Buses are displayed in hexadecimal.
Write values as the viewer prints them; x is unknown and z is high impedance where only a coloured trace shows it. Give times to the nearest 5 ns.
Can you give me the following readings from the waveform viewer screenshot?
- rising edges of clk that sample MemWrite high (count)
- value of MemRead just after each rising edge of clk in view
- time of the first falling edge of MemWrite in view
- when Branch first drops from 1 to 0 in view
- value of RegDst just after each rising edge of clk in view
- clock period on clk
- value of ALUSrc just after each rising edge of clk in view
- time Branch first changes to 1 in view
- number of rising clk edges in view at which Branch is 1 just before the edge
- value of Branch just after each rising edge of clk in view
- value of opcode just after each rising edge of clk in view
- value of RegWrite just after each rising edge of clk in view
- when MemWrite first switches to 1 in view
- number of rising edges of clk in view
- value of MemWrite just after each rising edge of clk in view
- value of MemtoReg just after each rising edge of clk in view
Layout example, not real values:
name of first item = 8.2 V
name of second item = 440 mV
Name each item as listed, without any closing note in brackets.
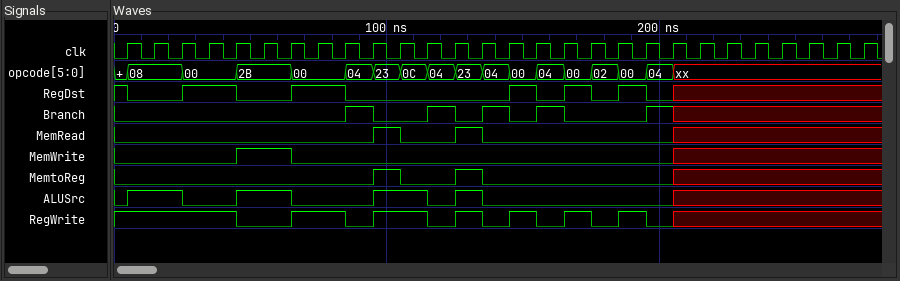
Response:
rising edges of clk that sample MemWrite high = 2
value of MemRead just after each rising edge of clk in view = 0 0 0 0 0 0 0 0 0 1 0 0 1 0 0 0 0 0 0 0 x x x x x x x x
time of the first falling edge of MemWrite in view = 65 ns
when Branch first drops from 1 to 0 in view = 95 ns
value of RegDst just after each rising edge of clk in view = 0 0 1 1 0 0 1 1 0 0 0 0 0 0 1 0 1 0 1 0 x x x x x x x x
clock period on clk = 10 ns
value of ALUSrc just after each rising edge of clk in view = 1 1 0 0 1 1 0 0 0 1 1 0 1 0 0 0 0 0 0 0 x x x x x x x x
time Branch first changes to 1 in view = 85 ns
number of rising clk edges in view at which Branch is 1 just before the edge = 5
value of Branch just after each rising edge of clk in view = 0 0 0 0 0 0 0 0 1 0 0 1 0 1 0 1 0 0 0 1 x x x x x x x x
value of opcode just after each rising edge of clk in view = 08, 08, 00, 00, 2B, 2B, 00, 00, 04, 23, 0C, 04, 23, 04, 00, 04, 00, 02, 00, 04, xx, xx, xx, xx, xx, xx, xx, xx
value of RegWrite just after each rising edge of clk in view = 1 1 1 1 0 0 1 1 0 1 1 0 1 0 1 0 1 0 1 0 x x x x x x x x
when MemWrite first switches to 1 in view = 45 ns
number of rising edges of clk in view = 28
value of MemWrite just after each rising edge of clk in view = 0 0 0 0 1 1 0 0 0 0 0 0 0 0 0 0 0 0 0 0 x x x x x x x x
value of MemtoReg just after each rising edge of clk in view = 0 0 0 0 0 0 0 0 0 1 0 0 1 0 0 0 0 0 0 0 x x x x x x x x
